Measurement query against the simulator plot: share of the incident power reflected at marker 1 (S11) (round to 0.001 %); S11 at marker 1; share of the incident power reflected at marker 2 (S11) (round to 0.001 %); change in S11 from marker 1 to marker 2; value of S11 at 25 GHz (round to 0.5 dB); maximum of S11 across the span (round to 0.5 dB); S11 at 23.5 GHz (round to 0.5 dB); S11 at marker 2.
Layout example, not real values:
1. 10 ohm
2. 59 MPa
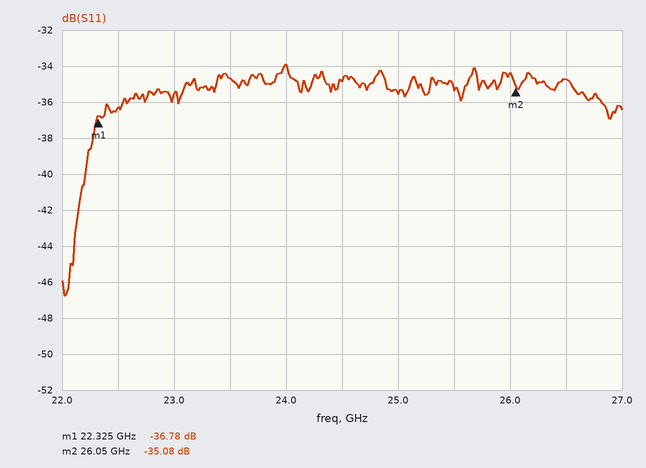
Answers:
1. 0.021 %
2. -36.78 dB
3. 0.031 %
4. 1.70 dB
5. -35.5 dB
6. -34.0 dB
7. -34.5 dB
8. -35.08 dB
